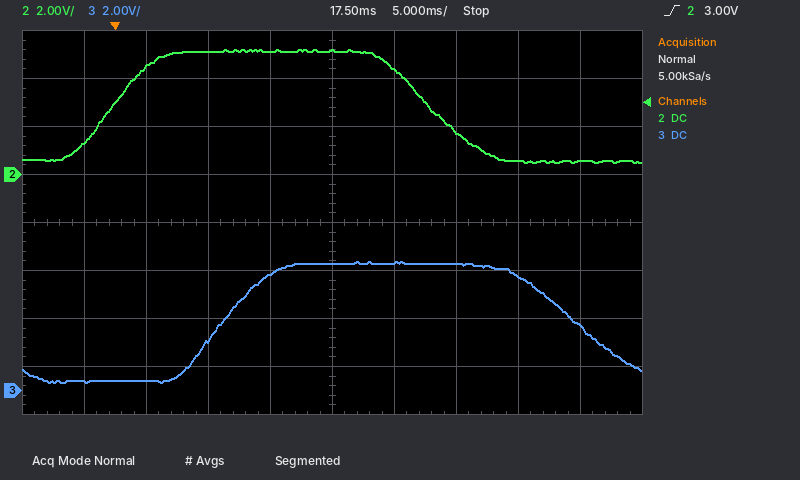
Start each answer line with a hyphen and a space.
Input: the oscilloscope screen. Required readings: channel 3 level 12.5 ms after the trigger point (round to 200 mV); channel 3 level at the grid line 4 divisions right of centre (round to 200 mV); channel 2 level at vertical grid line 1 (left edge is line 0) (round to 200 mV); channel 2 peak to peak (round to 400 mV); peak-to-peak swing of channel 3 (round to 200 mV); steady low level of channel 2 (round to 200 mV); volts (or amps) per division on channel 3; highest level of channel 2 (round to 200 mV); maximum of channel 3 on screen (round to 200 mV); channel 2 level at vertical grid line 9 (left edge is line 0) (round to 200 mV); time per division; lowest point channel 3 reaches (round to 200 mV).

- 4.8 V
- 2.8 V
- 1.4 V
- 4.8 V
- 5.0 V
- 600 mV
- 2 V
- 5.2 V
- 5.4 V
- 600 mV
- 5 ms
- 400 mV
